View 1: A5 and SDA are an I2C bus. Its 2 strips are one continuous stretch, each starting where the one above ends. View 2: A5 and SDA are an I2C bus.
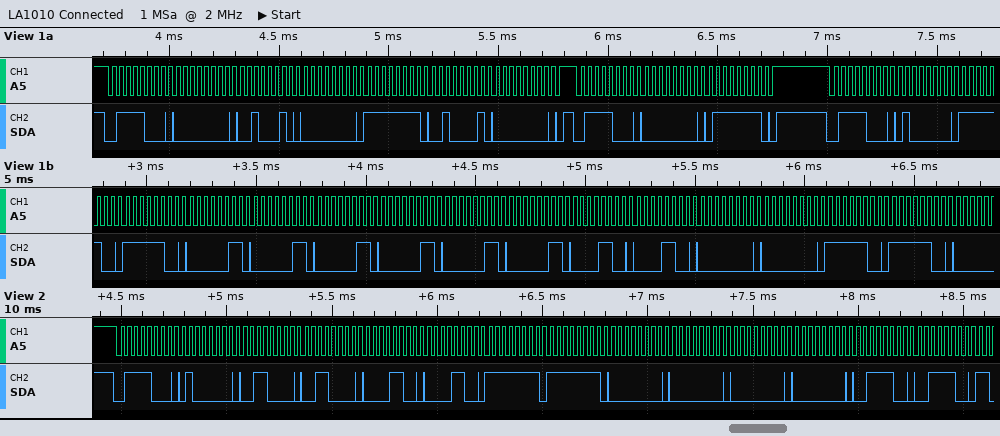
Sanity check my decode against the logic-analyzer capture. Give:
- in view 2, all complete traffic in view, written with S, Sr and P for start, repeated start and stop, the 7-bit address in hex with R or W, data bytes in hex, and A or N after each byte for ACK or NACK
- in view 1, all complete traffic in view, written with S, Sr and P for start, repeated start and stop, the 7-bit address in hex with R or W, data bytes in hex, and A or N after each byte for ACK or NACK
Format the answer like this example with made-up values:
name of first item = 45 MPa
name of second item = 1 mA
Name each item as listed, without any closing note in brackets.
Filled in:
in view 2, all complete traffic in view, written with S, Sr and P for start, repeated start and stop, the 7-bit address in hex with R or W, data bytes in hex, and A or N after each byte for ACK or NACK = S 3CW A 40 A 30 A 30 A 0C A 0C A FF A FF A 00 A 00 A 00 A 00 A 3C A 3C A
in view 1, all complete traffic in view, written with S, Sr and P for start, repeated start and stop, the 7-bit address in hex with R or W, data bytes in hex, and A or N after each byte for ACK or NACK = S 3CW A 00 A 22 A 00 A FF A 21 A 00 A P S 3CW A 00 A 7F A P S 3CW A 40 A FC A FC A 03 A 03 A 03 A 03 A 03 A 03 A 0C A 0C A 00 A 00 A FC A FC A
